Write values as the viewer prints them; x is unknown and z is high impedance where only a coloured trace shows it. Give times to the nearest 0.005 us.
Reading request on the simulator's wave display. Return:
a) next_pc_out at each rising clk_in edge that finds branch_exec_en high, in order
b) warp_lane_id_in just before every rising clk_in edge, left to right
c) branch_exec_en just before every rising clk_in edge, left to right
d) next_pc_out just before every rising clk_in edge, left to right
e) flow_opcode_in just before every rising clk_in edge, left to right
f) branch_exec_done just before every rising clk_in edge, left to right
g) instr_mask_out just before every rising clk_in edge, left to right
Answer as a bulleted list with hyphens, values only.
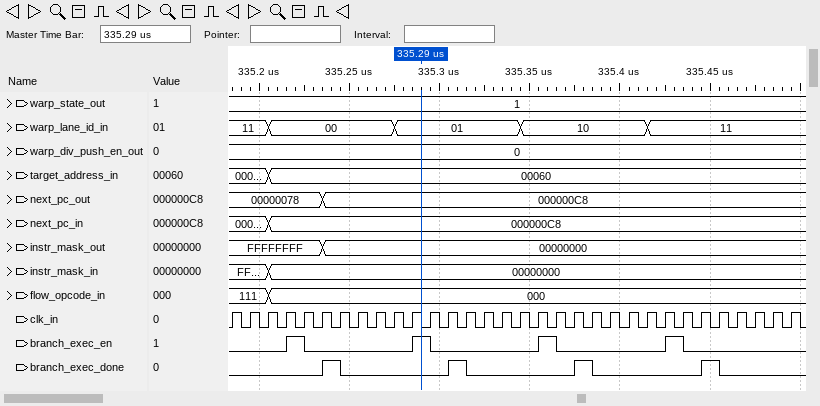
- 00000078, 000000C8, 000000C8, 000000C8
- 11, 11, 11, 00, 00, 00, 00, 00, 00, 00, 01, 01, 01, 01, 01, 01, 01, 10, 10, 10, 10, 10, 10, 10, 11, 11, 11, 11, 11, 11, 11, 11
- 0 0 0 0 1 0 0 0 0 0 0 1 0 0 0 0 0 0 1 0 0 0 0 0 0 1 0 0 0 0 0 0
- 00000078, 00000078, 00000078, 00000078, 00000078, 00000078, 000000C8, 000000C8, 000000C8, 000000C8, 000000C8, 000000C8, 000000C8, 000000C8, 000000C8, 000000C8, 000000C8, 000000C8, 000000C8, 000000C8, 000000C8, 000000C8, 000000C8, 000000C8, 000000C8, 000000C8, 000000C8, 000000C8, 000000C8, 000000C8, 000000C8, 000000C8
- 111, 111, 111, 000, 000, 000, 000, 000, 000, 000, 000, 000, 000, 000, 000, 000, 000, 000, 000, 000, 000, 000, 000, 000, 000, 000, 000, 000, 000, 000, 000, 000
- 0 0 0 0 0 0 1 0 0 0 0 0 0 1 0 0 0 0 0 0 1 0 0 0 0 0 0 1 0 0 0 0
- FFFFFFFF, FFFFFFFF, FFFFFFFF, FFFFFFFF, FFFFFFFF, FFFFFFFF, 00000000, 00000000, 00000000, 00000000, 00000000, 00000000, 00000000, 00000000, 00000000, 00000000, 00000000, 00000000, 00000000, 00000000, 00000000, 00000000, 00000000, 00000000, 00000000, 00000000, 00000000, 00000000, 00000000, 00000000, 00000000, 00000000
